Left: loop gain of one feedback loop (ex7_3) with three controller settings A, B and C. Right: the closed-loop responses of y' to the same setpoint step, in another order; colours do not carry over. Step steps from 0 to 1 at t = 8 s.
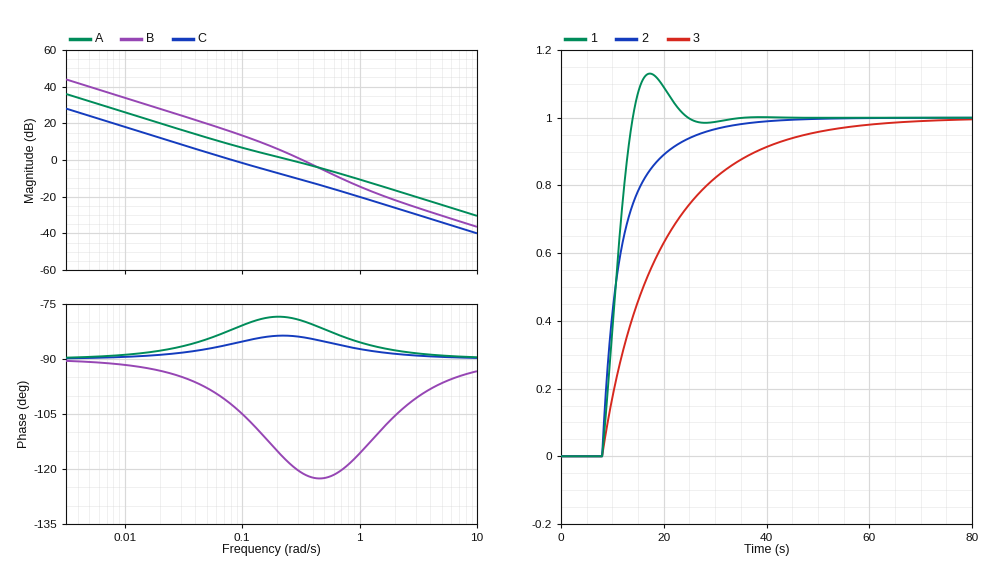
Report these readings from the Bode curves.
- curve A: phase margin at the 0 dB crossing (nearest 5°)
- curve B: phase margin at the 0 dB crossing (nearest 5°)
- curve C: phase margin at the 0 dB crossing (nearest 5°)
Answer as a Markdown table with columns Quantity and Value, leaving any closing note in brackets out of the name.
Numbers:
| Quantity | Value |
|---|---|
| curve A: phase margin at the 0 dB crossing | 100° |
| curve B: phase margin at the 0 dB crossing | 60° |
| curve C: phase margin at the 0 dB crossing | 95° |
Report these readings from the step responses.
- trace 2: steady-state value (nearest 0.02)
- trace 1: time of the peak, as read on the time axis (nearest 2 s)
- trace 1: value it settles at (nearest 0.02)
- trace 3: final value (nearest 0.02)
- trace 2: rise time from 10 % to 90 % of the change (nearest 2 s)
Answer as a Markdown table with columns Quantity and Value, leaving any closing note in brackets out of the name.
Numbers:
| Quantity | Value |
|---|---|
| trace 2: steady-state value | 1.00 |
| trace 1: time of the peak, as read on the time axis | 18 s |
| trace 1: value it settles at | 1.00 |
| trace 3: final value | 1.00 |
| trace 2: rise time from 10 % to 90 % of the change | 12 s |
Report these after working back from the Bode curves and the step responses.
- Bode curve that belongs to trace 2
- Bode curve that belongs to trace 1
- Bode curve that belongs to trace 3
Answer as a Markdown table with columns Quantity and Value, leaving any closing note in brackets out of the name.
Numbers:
| Quantity | Value |
|---|---|
| Bode curve that belongs to trace 2 | A |
| Bode curve that belongs to trace 1 | B |
| Bode curve that belongs to trace 3 | C |
